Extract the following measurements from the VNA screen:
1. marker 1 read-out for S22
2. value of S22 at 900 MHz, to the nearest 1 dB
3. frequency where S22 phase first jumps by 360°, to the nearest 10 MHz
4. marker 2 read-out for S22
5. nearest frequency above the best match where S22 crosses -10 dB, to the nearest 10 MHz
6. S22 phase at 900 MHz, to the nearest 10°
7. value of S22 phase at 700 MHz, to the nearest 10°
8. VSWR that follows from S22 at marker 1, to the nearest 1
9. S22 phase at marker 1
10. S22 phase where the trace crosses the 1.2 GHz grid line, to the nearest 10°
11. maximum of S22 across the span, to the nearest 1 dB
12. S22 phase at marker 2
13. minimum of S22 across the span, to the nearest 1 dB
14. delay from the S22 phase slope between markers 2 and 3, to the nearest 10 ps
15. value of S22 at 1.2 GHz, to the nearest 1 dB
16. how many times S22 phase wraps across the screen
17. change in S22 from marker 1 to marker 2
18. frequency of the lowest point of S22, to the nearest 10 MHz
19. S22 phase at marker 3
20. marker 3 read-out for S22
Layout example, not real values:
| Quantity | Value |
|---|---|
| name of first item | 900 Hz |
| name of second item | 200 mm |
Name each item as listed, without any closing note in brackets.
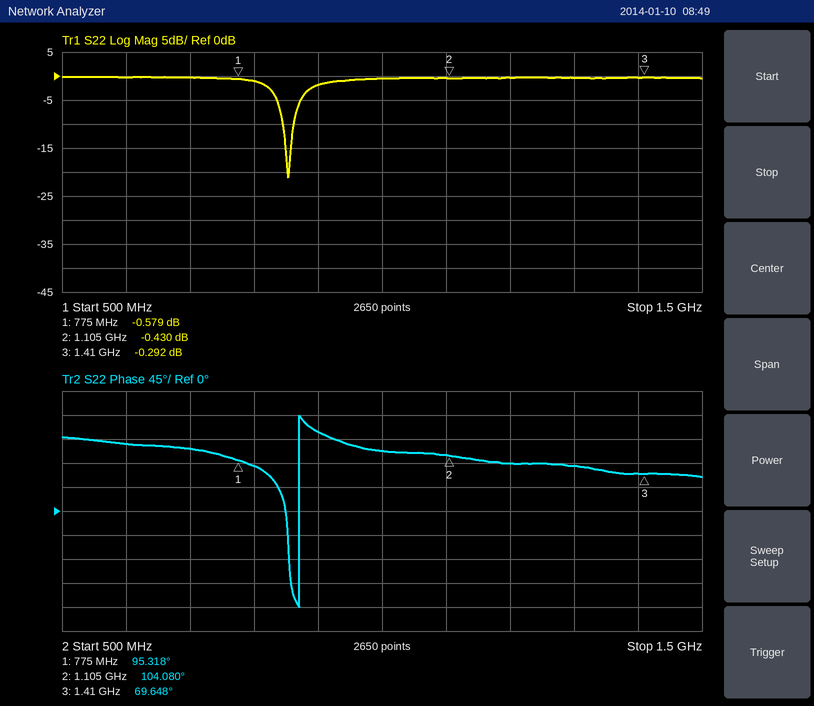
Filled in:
| Quantity | Value |
|---|---|
| marker 1 read-out for S22 | -0.579 dB |
| value of S22 at 900 MHz, to the nearest 1 dB | -2 dB |
| frequency where S22 phase first jumps by 360°, to the nearest 10 MHz | 870 MHz |
| marker 2 read-out for S22 | -0.430 dB |
| nearest frequency above the best match where S22 crosses -10 dB, to the nearest 10 MHz | 860 MHz |
| S22 phase at 900 MHz, to the nearest 10° | 150° |
| value of S22 phase at 700 MHz, to the nearest 10° | 120° |
| VSWR that follows from S22 at marker 1, to the nearest 1 | 30 |
| S22 phase at marker 1 | 95.318° |
| S22 phase where the trace crosses the 1.2 GHz grid line, to the nearest 10° | 90° |
| maximum of S22 across the span, to the nearest 1 dB | 0 dB |
| S22 phase at marker 2 | 104.080° |
| minimum of S22 across the span, to the nearest 1 dB | -21 dB |
| delay from the S22 phase slope between markers 2 and 3, to the nearest 10 ps | 310 ps |
| value of S22 at 1.2 GHz, to the nearest 1 dB | 0 dB |
| how many times S22 phase wraps across the screen | 1 |
| change in S22 from marker 1 to marker 2 | 0.149 dB |
| frequency of the lowest point of S22, to the nearest 10 MHz | 850 MHz |
| S22 phase at marker 3 | 69.648° |
| marker 3 read-out for S22 | -0.292 dB |
